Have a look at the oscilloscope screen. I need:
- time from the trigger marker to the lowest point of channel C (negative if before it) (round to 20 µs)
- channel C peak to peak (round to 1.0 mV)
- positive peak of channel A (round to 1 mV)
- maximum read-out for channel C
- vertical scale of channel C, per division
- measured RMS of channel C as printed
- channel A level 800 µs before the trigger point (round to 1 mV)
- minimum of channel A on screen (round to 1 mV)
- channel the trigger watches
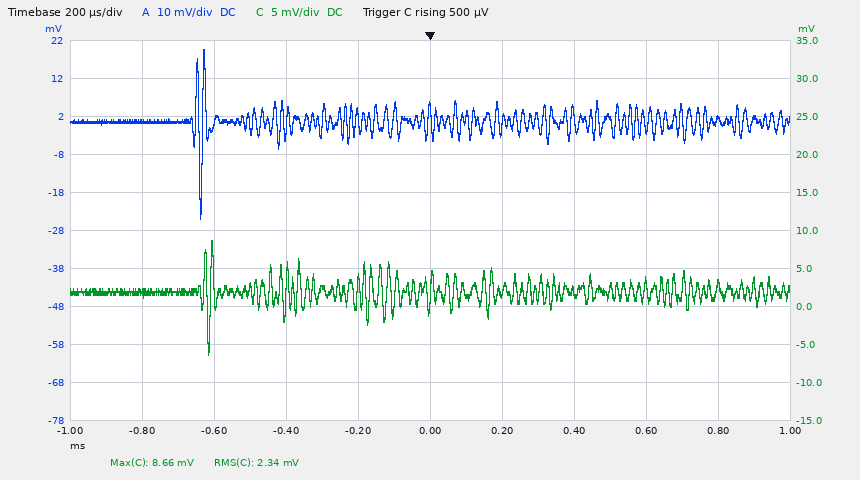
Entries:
-620 µs
15.0 mV
20 mV
8.66 mV
5 mV
2.34 mV
1 mV
-25 mV
channel C
